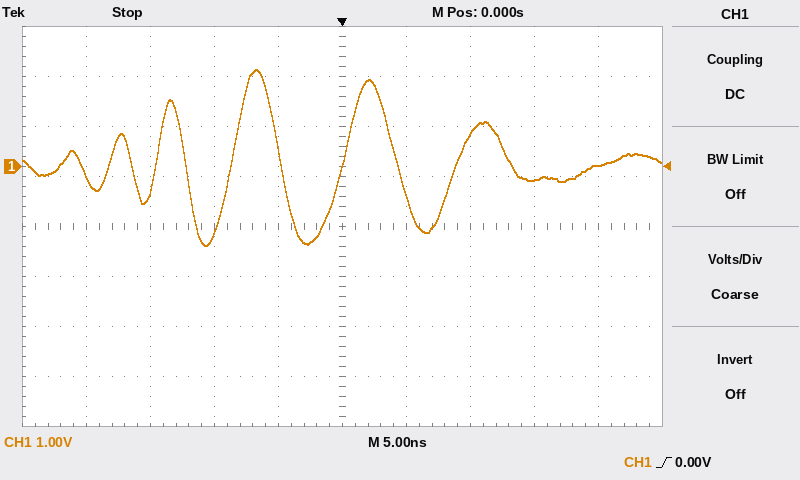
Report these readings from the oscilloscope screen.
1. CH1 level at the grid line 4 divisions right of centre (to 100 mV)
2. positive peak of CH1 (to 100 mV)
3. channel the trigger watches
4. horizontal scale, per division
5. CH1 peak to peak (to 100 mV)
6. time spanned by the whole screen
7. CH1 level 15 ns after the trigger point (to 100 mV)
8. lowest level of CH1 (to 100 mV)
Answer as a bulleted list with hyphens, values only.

- 0.0 V
- 1.9 V
- CH1
- 5 ns
- 3.5 V
- 50 ns
- -300 mV
- -1.6 V
